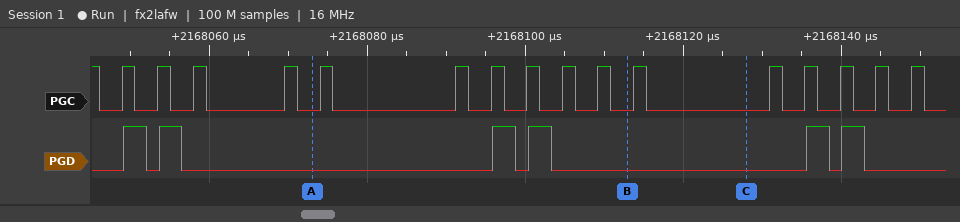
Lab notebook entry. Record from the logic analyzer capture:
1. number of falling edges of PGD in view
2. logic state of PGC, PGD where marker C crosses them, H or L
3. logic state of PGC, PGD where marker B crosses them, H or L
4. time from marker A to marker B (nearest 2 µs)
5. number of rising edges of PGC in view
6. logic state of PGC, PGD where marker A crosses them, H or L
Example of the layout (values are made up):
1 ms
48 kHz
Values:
6
PGC=L, PGD=L
PGC=L, PGD=L
40 µs
16
PGC=L, PGD=L
